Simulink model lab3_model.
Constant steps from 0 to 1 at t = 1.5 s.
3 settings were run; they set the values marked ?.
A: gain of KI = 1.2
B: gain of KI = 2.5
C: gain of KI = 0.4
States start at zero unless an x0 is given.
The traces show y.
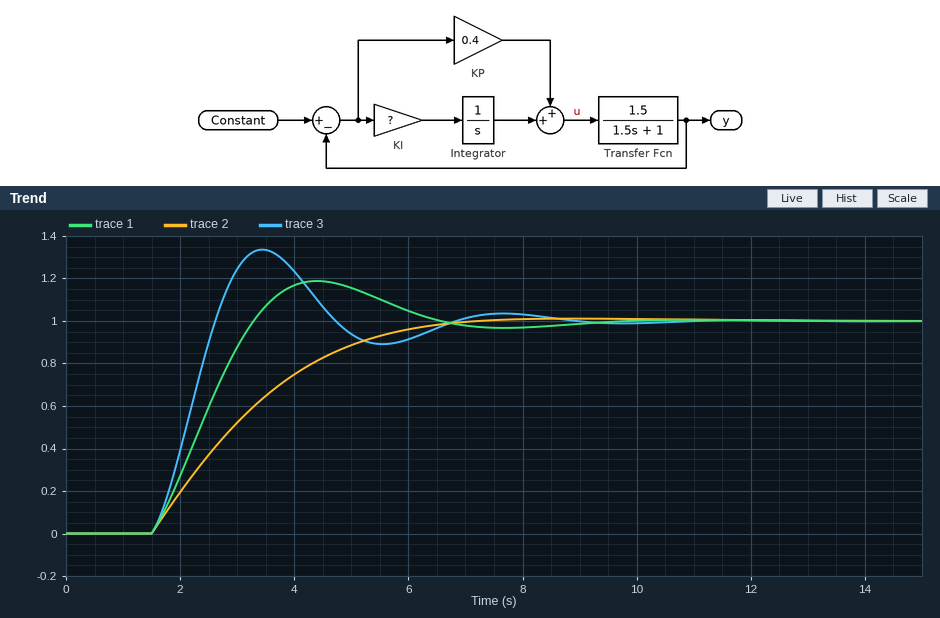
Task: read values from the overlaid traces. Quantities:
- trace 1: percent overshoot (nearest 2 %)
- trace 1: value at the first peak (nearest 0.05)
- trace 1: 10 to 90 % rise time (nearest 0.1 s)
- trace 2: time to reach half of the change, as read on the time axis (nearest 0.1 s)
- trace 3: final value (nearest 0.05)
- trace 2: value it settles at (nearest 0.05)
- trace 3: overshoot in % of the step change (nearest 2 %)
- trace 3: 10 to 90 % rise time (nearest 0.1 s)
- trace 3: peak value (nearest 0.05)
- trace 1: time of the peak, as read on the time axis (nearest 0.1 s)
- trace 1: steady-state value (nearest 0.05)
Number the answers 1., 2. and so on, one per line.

1. 18 %
2. 1.20
3. 1.3 s
4. 2.9 s
5. 1.00
6. 1.00
7. 34 %
8. 0.8 s
9. 1.35
10. 4.4 s
11. 1.00
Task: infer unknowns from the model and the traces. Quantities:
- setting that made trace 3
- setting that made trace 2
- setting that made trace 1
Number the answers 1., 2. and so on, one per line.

1. B
2. C
3. A
